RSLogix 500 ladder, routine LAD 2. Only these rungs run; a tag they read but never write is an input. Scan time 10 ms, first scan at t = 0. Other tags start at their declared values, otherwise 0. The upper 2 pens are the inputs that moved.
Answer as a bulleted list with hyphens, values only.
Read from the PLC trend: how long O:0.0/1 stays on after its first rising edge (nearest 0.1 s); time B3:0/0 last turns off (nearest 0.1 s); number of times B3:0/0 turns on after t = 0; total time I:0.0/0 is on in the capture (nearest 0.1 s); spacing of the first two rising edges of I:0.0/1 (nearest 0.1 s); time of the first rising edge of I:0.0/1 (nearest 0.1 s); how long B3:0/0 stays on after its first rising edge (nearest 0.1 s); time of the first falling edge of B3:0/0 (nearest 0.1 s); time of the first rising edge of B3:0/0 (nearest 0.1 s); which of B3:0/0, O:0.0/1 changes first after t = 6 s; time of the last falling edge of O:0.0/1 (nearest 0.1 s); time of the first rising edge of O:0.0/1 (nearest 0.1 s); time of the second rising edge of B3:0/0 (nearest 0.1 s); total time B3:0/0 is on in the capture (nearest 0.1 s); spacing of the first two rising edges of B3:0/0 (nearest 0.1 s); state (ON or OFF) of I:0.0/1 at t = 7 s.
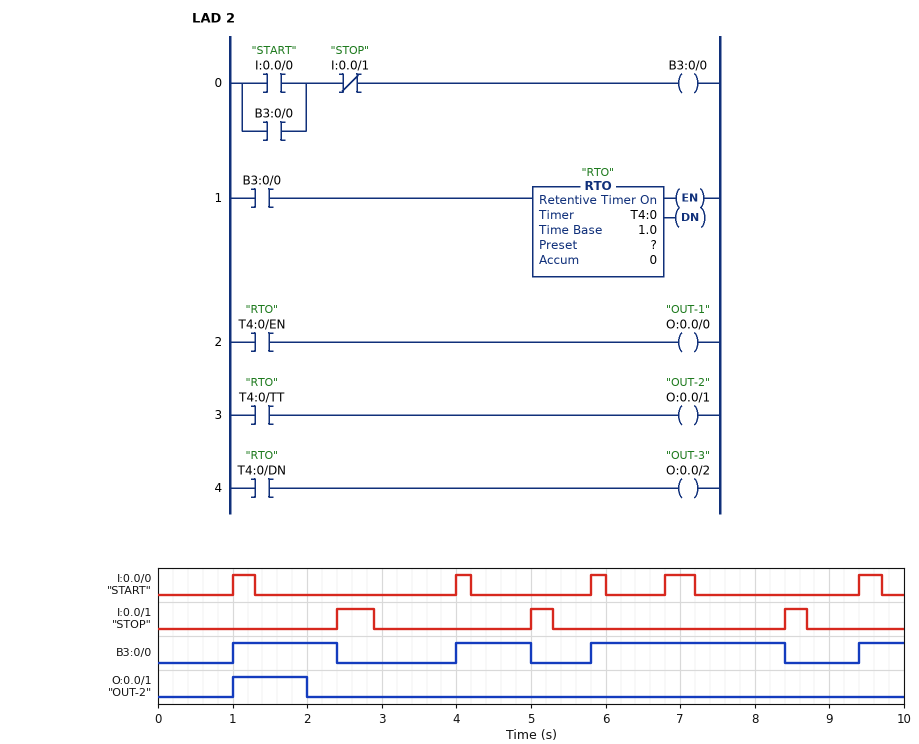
- 1.0 s
- 8.4 s
- 4
- 1.4 s
- 2.6 s
- 2.4 s
- 1.4 s
- 2.4 s
- 1.0 s
- B3:0/0
- 2.0 s
- 1.0 s
- 4.0 s
- 5.6 s
- 3.0 s
- OFF
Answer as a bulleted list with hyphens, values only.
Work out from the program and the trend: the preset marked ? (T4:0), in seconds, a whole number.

- 1 s
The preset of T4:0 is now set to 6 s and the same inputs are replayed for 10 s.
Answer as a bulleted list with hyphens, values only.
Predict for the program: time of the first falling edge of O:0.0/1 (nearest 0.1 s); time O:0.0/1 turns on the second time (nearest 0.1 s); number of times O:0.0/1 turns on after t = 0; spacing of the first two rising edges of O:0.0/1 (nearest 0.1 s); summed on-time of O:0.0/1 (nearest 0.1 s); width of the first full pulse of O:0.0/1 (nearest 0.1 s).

- 2.4 s
- 4.0 s
- 4
- 3.0 s
- 5.6 s
- 1.4 s
